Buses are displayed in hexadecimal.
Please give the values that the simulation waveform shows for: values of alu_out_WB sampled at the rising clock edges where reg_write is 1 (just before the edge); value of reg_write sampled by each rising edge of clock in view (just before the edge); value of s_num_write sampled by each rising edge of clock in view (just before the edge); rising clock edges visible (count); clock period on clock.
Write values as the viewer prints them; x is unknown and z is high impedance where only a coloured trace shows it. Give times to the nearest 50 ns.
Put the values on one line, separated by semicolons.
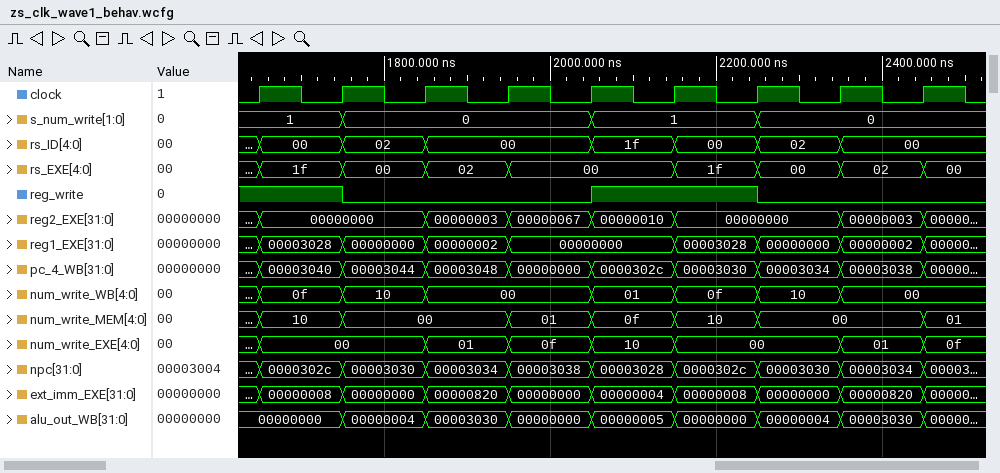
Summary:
00000000, 00000000, 00000005, 00000000; 1 1 0 0 0 1 1 0 0; 1, 1, 0, 0, 0, 1, 1, 0, 0; 9; 100 ns
